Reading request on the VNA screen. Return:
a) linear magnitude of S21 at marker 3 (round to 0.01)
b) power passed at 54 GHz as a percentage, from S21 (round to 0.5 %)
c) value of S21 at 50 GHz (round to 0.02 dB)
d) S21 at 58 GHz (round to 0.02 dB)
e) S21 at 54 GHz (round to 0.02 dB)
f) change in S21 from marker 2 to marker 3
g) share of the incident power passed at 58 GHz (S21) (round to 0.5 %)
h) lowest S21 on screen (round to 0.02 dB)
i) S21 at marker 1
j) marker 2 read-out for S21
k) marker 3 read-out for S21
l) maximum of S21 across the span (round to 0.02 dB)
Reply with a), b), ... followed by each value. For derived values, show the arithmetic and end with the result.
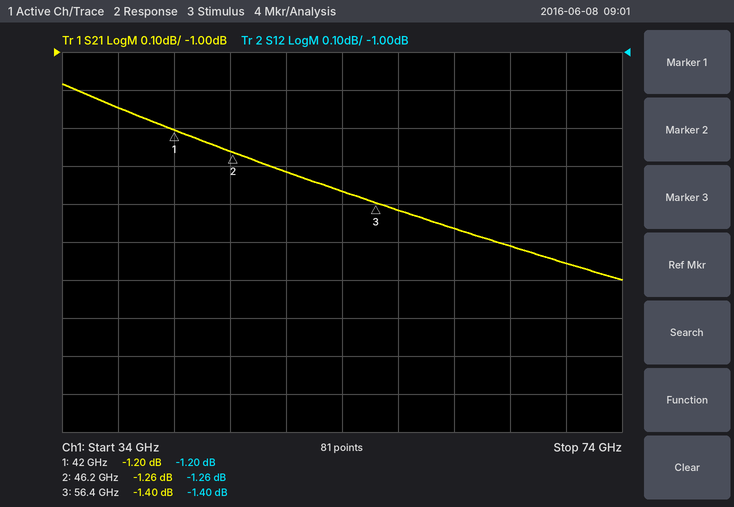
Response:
a) 10^(-1.4/20) ≈ 0.85
b) 10^(-1.36/10) ≈ 73.1 %, so 73.0 % to the nearest 0.5 %
c) -1.32 dB
d) -1.42 dB
e) -1.36 dB
f) -1.4 − (-1.26) = -0.14 dB
g) 10^(-1.42/10) ≈ 72.1 %, so 72.0 % to the nearest 0.5 %
h) -1.60 dB
i) -1.20 dB
j) -1.26 dB
k) -1.40 dB
l) -1.08 dB
